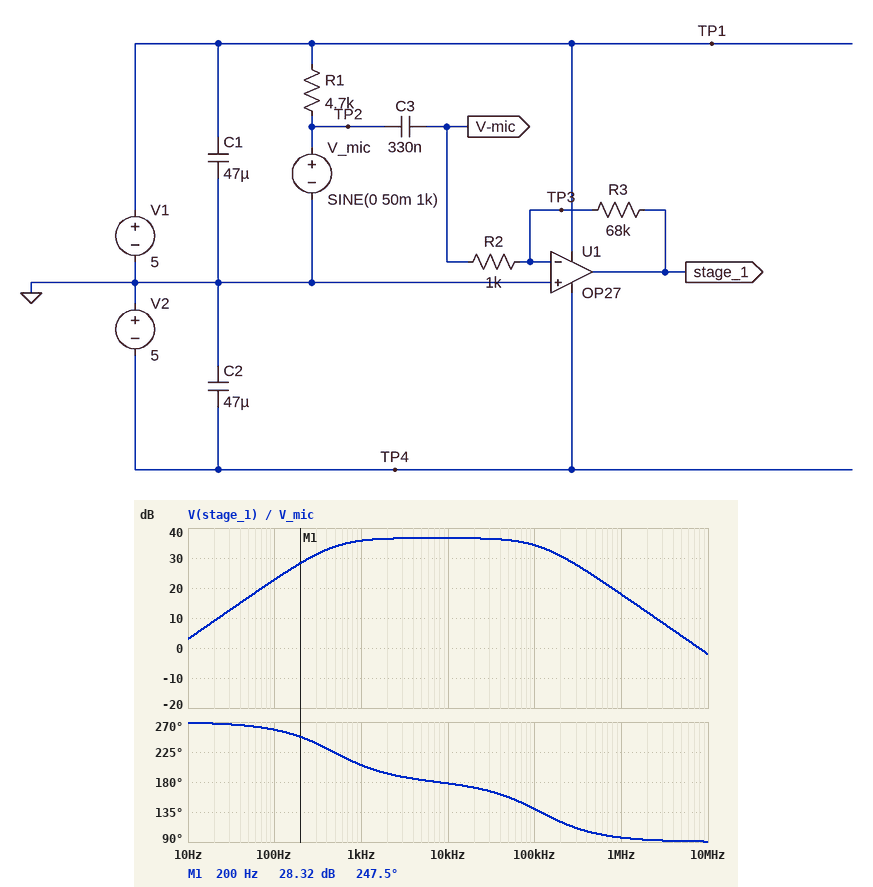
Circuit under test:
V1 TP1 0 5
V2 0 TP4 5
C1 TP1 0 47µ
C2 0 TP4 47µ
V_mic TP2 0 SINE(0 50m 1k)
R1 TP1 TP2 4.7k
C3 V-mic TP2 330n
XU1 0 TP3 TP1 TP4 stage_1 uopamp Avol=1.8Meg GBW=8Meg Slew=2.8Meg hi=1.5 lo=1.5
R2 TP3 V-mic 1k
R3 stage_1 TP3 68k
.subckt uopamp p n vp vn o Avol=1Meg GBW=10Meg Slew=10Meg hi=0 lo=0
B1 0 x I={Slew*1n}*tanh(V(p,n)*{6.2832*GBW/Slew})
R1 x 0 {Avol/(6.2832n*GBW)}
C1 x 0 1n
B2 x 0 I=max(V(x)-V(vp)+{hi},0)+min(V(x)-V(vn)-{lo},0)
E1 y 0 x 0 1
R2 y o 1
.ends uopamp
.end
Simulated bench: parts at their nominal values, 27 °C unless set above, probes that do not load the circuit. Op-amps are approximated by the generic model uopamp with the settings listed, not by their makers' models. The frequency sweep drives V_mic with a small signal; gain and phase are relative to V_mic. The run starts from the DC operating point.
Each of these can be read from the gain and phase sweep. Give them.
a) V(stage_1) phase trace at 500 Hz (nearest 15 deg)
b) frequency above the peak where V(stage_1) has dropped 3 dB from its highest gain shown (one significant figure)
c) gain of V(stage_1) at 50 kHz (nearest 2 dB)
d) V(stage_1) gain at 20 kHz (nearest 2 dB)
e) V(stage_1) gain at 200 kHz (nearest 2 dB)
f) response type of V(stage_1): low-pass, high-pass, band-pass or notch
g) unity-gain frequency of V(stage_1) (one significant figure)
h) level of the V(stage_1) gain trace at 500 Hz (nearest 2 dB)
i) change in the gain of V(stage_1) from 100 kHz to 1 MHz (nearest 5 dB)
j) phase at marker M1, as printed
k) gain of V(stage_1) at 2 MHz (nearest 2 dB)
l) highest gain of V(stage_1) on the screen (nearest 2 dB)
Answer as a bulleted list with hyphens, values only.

- 225 deg
- 100 kHz
- 36 dB
- 36 dB
- 30 dB
- band-pass
- 8 MHz
- 34 dB
- -15 dB
- 247.5 deg
- 12 dB
- 36 dB
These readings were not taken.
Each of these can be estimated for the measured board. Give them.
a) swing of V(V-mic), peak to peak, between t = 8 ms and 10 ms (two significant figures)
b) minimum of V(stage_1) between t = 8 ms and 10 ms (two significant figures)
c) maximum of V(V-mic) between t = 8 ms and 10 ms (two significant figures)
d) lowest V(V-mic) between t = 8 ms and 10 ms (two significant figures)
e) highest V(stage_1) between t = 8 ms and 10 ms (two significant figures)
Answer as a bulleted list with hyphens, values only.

- 90 mV
- -3.1 V
- 45 mV
- -45 mV
- 3.1 V
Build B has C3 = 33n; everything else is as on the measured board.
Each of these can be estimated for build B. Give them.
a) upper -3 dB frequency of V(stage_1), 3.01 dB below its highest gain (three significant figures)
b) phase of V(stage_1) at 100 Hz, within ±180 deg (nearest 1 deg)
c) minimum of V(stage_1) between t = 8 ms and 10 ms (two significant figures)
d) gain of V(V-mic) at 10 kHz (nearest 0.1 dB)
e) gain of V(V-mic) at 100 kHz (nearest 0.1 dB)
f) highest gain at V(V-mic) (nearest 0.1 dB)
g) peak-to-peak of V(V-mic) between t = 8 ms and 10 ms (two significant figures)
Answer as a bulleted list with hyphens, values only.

- 121 kHz
- -91 deg
- -690 mV
- -0.6 dB
- 0.2 dB
- 0.3 dB
- 20 mV
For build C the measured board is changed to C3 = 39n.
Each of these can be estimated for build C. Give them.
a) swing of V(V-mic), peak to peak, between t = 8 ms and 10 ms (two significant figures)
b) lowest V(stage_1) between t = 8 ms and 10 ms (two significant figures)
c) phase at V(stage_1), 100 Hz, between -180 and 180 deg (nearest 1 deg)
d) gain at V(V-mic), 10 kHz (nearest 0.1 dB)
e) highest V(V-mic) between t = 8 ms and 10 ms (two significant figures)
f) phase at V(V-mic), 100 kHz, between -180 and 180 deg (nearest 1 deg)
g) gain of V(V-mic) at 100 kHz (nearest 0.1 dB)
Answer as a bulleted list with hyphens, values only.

- 24 mV
- -810 mV
- -91 deg
- -0.4 dB
- 12 mV
- 1 deg
- 0.2 dB
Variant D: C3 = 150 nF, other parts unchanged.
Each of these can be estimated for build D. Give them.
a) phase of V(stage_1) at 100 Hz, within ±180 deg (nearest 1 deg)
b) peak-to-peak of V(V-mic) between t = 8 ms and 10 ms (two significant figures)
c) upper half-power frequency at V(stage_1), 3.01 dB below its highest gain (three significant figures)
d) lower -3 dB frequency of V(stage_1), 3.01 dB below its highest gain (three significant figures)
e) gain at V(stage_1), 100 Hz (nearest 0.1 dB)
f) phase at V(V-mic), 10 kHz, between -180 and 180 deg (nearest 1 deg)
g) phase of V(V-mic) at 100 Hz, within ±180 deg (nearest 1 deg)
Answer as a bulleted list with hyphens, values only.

- -95 deg
- 69 mV
- 117 kHz
- 1.05 kHz
- 16.1 dB
- 6 deg
- 85 deg
